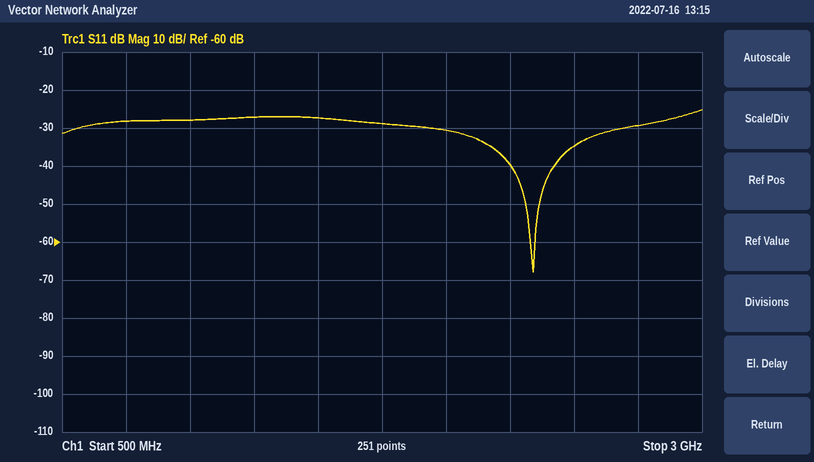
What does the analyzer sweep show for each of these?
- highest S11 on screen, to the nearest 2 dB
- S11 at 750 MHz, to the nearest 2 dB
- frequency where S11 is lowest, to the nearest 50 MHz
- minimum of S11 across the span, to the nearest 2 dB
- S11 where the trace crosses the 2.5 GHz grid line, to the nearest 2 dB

-26 dB
-28 dB
2.35 GHz
-68 dB
-34 dB
